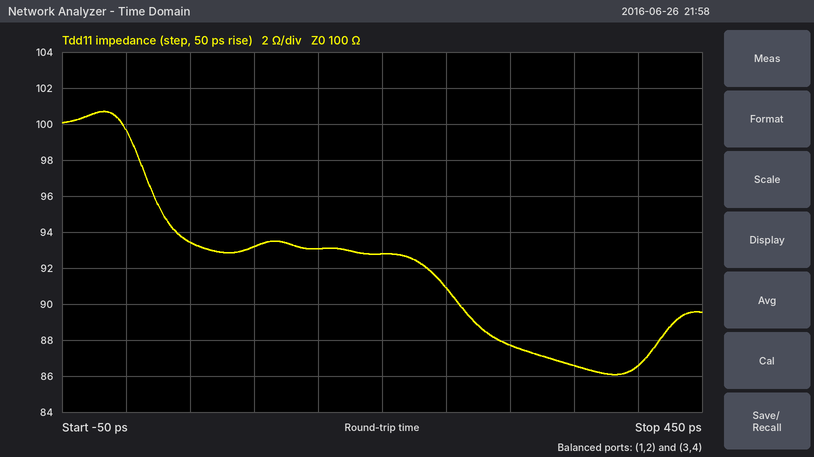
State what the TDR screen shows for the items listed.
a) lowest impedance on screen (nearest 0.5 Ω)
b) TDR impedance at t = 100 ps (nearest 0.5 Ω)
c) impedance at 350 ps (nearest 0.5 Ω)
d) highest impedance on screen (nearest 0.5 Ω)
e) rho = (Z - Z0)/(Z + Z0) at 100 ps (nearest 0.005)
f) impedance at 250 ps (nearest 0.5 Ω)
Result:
86.0 Ω
93.0 Ω
86.5 Ω
100.5 Ω
-0.035
91.0 Ω
